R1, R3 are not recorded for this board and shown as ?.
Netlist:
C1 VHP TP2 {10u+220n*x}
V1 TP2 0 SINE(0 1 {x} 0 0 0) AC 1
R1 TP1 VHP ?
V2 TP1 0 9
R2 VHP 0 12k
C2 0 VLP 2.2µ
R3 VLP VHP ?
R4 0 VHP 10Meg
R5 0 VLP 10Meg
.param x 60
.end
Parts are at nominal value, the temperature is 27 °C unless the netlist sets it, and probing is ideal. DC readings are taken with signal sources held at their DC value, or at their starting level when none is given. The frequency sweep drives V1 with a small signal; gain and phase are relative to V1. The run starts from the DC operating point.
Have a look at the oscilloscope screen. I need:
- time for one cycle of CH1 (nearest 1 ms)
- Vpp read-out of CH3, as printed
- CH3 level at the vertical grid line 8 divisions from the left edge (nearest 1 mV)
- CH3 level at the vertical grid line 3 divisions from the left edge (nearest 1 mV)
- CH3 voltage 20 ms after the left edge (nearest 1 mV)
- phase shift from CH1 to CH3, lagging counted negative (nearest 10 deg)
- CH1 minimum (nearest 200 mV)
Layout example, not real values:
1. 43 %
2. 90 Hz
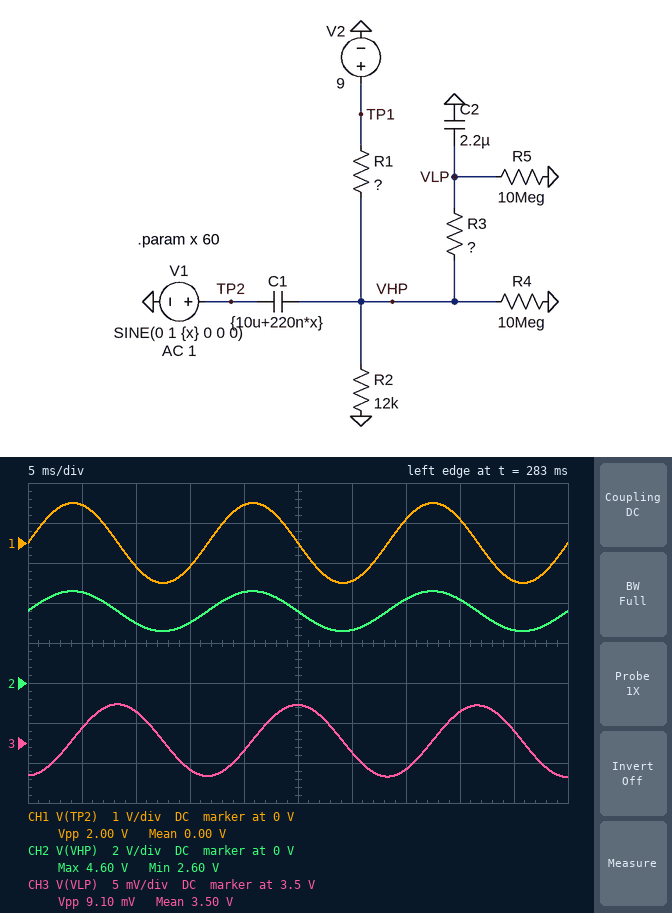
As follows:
1. 17 ms
2. 9.10 mV
3. 3.504 V
4. 3.497 V
5. 3.499 V
6. -90 deg
7. -1.0 V
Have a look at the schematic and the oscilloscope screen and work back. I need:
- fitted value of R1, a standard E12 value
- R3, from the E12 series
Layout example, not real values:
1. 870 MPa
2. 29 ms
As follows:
1. 18 kΩ
2. 270 kΩ
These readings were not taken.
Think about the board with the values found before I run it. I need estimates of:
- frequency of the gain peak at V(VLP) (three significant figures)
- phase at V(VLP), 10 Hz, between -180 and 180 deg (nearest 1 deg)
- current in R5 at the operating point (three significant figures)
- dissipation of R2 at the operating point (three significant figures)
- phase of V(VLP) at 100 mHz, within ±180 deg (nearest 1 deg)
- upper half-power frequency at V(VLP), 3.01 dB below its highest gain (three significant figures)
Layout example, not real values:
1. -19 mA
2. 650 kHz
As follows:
1. 512 mHz
2. -83 deg
3. 350 nA
4. 1.08 mW
5. 64 deg
6. 1.44 Hz
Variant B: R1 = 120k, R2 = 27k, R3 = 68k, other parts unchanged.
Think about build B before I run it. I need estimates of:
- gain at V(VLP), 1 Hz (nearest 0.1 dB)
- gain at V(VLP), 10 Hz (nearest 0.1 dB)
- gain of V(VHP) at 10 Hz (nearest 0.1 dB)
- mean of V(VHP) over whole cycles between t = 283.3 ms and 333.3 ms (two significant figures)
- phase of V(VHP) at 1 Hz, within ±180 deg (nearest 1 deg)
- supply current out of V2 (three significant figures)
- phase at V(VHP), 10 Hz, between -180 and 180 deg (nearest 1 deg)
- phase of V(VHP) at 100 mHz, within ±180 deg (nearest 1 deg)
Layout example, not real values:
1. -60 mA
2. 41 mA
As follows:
1. -3.7 dB
2. -19.5 dB
3. 0 dB
4. 1.6 V
5. 19 deg
6. 61.3 µA
7. 2 deg
8. 71 deg
